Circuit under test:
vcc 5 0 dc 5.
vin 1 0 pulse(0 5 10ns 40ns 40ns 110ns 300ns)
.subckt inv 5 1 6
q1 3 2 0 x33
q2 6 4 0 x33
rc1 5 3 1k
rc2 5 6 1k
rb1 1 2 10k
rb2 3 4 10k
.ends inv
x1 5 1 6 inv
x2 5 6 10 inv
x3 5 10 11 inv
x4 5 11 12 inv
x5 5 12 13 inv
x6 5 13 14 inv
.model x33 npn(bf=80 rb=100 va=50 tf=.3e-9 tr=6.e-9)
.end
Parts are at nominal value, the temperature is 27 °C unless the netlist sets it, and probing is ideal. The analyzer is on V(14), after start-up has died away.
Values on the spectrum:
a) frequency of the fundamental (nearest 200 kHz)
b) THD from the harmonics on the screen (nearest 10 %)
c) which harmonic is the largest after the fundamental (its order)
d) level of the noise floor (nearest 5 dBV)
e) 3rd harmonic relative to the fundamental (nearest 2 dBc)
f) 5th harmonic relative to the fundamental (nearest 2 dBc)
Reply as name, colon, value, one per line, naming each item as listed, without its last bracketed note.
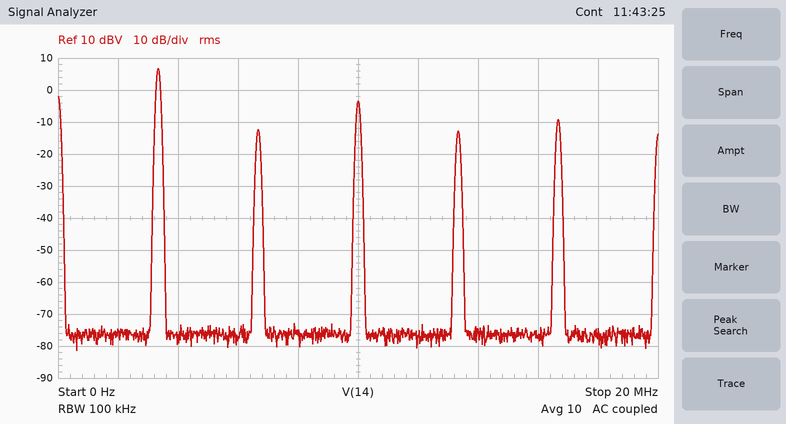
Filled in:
frequency of the fundamental: 3.4 MHz
THD from the harmonics on the screen: 40 %
which harmonic is the largest after the fundamental: 3
level of the noise floor: -75 dBV
3rd harmonic relative to the fundamental: -10 dBc
5th harmonic relative to the fundamental: -16 dBc
